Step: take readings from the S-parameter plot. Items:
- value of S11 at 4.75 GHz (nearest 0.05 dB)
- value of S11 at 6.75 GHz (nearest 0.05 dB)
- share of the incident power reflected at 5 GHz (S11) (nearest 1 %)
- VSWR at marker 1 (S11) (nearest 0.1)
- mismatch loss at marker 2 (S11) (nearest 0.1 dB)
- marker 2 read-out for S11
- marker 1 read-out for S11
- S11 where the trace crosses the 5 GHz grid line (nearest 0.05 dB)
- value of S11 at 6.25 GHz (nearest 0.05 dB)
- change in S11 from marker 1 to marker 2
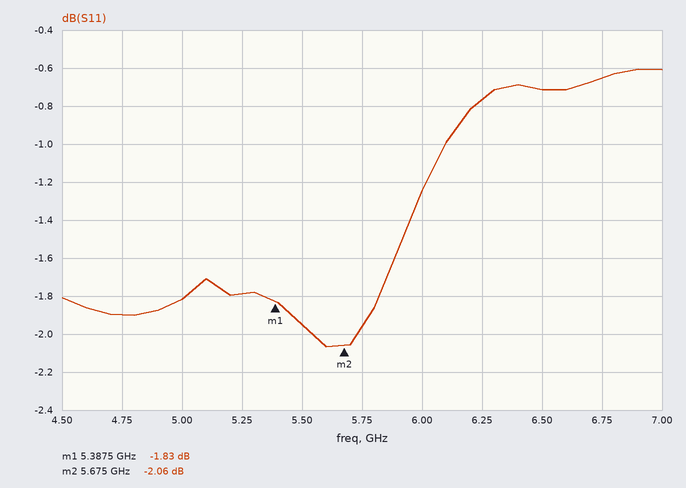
-1.90 dB
-0.65 dB
66 %
9.5
4.2 dB
-2.06 dB
-1.83 dB
-1.80 dB
-0.75 dB
-0.23 dB
